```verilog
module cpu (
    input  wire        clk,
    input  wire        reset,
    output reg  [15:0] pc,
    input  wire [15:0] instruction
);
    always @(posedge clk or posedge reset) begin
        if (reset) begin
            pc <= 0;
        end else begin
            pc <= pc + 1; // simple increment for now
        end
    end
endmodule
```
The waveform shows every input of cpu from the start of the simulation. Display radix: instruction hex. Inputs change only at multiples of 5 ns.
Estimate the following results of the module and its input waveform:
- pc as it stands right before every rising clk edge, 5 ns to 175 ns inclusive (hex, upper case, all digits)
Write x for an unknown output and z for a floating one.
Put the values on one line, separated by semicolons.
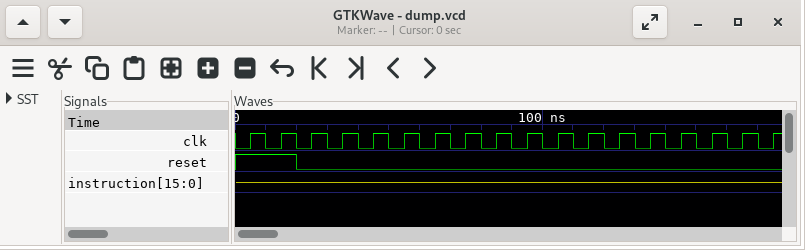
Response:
0000, 0000, 0000, 0001, 0002, 0003, 0004, 0005, 0006, 0007, 0008, 0009, 000A, 000B, 000C, 000D, 000E, 000F
